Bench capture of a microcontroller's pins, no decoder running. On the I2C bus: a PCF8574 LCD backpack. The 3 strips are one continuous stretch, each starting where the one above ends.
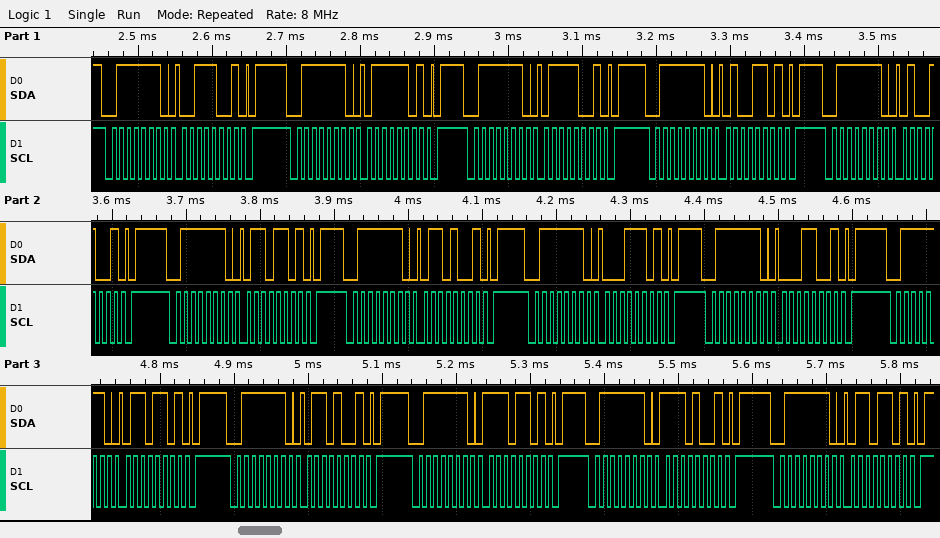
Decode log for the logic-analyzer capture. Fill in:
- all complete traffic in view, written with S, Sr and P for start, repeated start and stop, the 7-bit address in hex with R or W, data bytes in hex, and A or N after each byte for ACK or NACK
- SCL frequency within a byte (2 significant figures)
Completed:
S 3FW A 39 A P S 3FW A 7D A P S 3FW A 79 A P S 3FW A 4D A P S 3FW A 49 A P S 3FW A 6D A P S 3FW A 69 A P S 3FW A 1D A P S 3FW A 19 A P S 3FW A 6D A P S 3FW A 69 A P S 3FW A ED A P S 3FW A E9 A P S 3FW A 6D A P
100 kHz
